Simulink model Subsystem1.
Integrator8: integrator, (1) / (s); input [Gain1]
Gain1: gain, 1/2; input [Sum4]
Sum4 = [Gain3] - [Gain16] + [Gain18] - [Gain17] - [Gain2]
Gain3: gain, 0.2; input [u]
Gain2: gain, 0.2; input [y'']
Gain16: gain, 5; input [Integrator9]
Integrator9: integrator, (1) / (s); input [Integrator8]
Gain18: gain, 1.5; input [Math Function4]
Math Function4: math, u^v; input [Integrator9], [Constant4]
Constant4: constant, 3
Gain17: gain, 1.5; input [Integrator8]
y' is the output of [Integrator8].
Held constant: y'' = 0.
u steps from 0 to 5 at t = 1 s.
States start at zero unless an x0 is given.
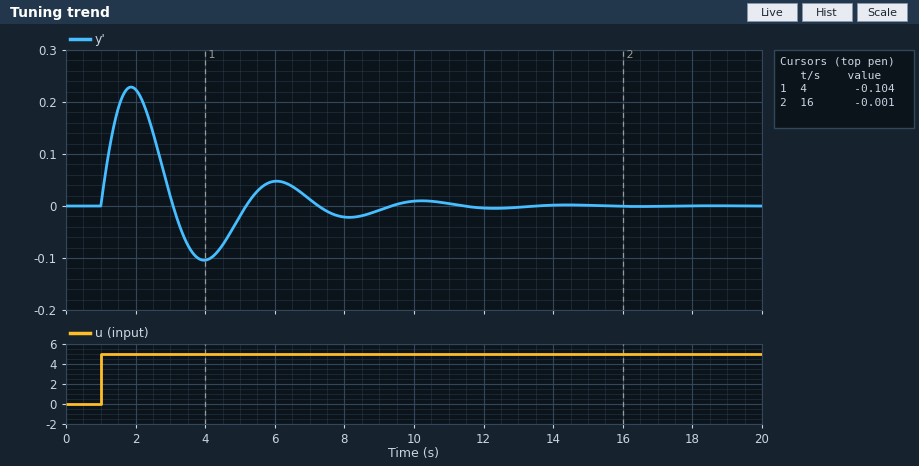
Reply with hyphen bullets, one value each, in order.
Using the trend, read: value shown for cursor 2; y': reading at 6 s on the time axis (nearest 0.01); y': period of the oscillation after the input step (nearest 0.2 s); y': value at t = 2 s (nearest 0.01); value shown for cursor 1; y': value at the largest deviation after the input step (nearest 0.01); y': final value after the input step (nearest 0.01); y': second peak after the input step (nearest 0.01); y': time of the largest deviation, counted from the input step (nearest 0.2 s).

- -0.001
- 0.05
- 4.2 s
- 0.22
- -0.104
- 0.23
- 0.00
- 0.05
- 0.8 s
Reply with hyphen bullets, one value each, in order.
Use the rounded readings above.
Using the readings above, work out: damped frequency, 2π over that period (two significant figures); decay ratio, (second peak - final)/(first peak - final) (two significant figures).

- 1.5 rad/s
- 0.22
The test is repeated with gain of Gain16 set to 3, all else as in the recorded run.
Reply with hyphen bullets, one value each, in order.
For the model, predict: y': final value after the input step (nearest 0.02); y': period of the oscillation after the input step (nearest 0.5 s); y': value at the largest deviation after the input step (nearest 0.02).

- 0.00
- 6.0 s
- 0.28
